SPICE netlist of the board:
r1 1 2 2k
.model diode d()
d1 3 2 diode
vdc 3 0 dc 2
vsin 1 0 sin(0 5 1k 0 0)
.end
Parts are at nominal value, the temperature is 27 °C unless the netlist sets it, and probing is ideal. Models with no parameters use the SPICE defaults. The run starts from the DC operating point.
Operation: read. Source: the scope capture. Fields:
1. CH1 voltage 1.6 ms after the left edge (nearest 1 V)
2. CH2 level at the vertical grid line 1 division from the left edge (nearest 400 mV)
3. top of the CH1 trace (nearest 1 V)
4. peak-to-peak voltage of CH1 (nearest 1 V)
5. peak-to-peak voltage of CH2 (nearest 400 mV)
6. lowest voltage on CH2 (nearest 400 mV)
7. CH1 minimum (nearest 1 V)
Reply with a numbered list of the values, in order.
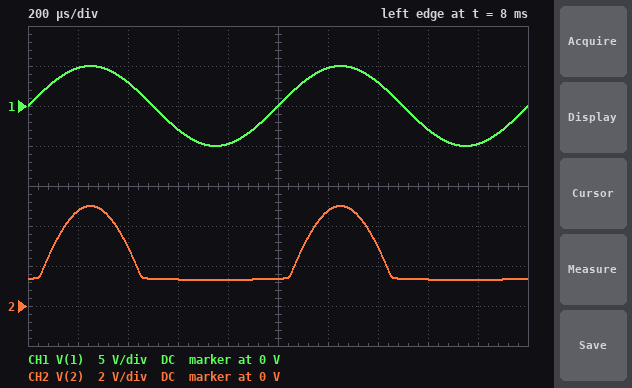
1. -3 V
2. 4.8 V
3. 5 V
4. 10 V
5. 3.6 V
6. 1.2 V
7. -5 V
